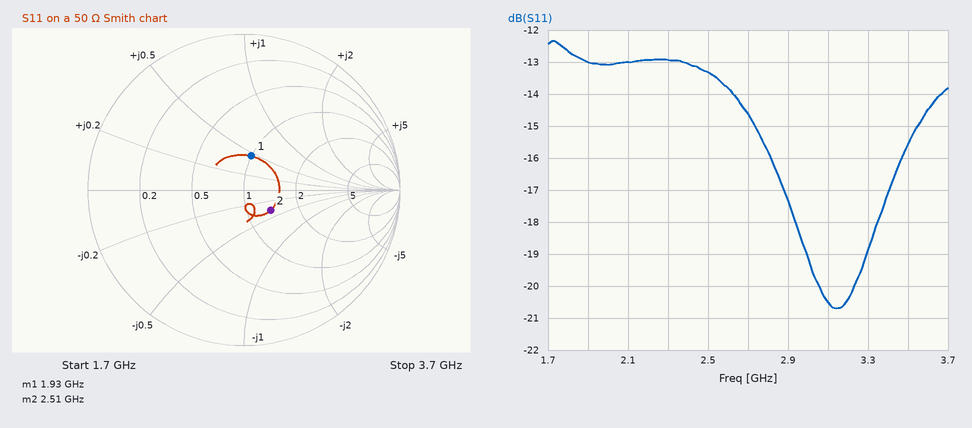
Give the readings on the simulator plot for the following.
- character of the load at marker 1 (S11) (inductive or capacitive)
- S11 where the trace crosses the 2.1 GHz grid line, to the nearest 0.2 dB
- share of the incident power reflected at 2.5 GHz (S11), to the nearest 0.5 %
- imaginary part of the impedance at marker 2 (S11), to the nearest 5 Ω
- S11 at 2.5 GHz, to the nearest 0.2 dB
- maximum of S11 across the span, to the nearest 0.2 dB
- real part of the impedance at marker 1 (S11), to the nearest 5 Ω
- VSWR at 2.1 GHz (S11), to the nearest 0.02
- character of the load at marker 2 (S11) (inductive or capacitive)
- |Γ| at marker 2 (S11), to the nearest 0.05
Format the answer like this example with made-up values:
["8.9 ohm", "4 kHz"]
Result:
["inductive", "-13.0 dB", "4.5 %", "-20 Ω", "-13.4 dB", "-12.4 dB", "50 Ω", "1.58", "capacitive", "0.20"]
